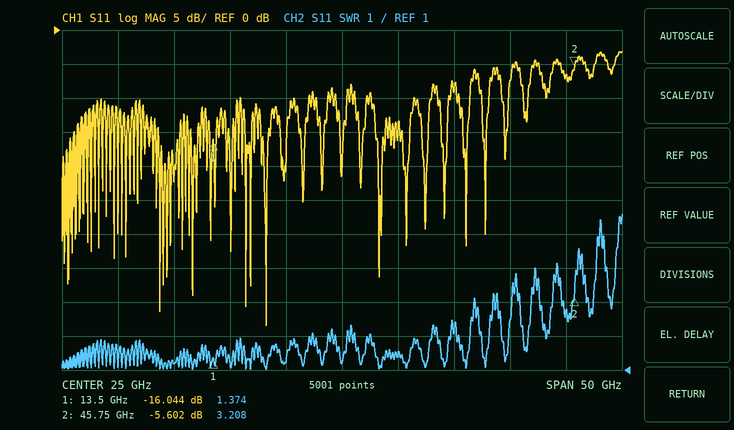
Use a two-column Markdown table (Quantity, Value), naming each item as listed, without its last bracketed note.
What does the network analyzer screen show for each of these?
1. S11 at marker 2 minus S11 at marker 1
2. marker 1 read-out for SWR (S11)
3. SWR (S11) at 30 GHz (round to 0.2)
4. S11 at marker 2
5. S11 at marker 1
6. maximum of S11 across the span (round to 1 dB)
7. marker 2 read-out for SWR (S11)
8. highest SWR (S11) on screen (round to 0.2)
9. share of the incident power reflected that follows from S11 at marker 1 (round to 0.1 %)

| Quantity | Value |
|---|---|
| S11 at marker 2 minus S11 at marker 1 | 10.442 dB |
| marker 1 read-out for SWR | 1.374 |
| SWR (S11) at 30 GHz | 1.4 |
| S11 at marker 2 | -5.602 dB |
| S11 at marker 1 | -16.044 dB |
| maximum of S11 across the span | -3 dB |
| marker 2 read-out for SWR | 3.208 |
| highest SWR (S11) on screen | 5.6 |
| share of the incident power reflected that follows from S11 at marker 1 | 2.5 % |
